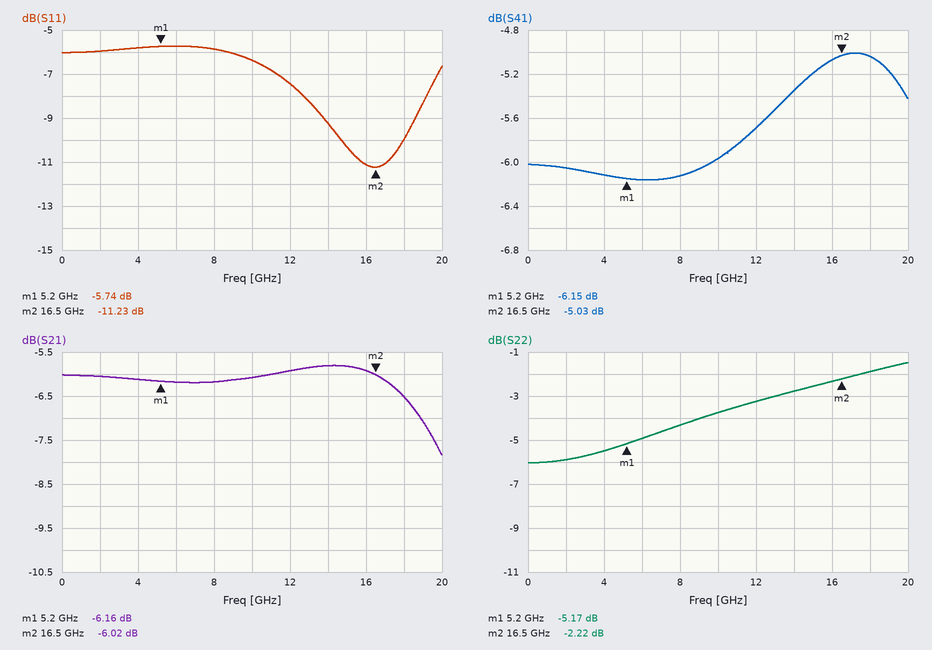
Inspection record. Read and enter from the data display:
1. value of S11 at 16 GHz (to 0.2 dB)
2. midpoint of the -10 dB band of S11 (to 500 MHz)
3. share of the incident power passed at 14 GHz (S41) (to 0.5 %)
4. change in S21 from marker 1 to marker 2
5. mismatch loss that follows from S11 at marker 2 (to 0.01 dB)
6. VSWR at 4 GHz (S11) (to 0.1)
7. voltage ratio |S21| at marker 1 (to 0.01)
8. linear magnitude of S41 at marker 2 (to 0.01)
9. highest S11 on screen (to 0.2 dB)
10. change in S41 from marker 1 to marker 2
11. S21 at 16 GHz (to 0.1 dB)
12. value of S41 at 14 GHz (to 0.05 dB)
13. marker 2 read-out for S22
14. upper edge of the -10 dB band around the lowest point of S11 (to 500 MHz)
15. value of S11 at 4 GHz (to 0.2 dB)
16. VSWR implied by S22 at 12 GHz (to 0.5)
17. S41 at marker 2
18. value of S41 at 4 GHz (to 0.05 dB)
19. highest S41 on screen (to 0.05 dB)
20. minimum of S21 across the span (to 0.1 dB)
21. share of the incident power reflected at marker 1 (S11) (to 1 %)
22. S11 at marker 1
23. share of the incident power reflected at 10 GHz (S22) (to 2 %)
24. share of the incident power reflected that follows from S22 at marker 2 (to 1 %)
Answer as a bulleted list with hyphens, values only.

- -11.2 dB
- 16.5 GHz
- 29.0 %
- 0.14 dB
- 0.34 dB
- 3.1
- 0.49
- 0.56
- -5.8 dB
- 1.12 dB
- -5.9 dB
- -5.35 dB
- -2.22 dB
- 18.0 GHz
- -5.8 dB
- 5.5
- -5.03 dB
- -6.10 dB
- -5.00 dB
- -7.8 dB
- 27 %
- -5.74 dB
- 42 %
- 60 %
